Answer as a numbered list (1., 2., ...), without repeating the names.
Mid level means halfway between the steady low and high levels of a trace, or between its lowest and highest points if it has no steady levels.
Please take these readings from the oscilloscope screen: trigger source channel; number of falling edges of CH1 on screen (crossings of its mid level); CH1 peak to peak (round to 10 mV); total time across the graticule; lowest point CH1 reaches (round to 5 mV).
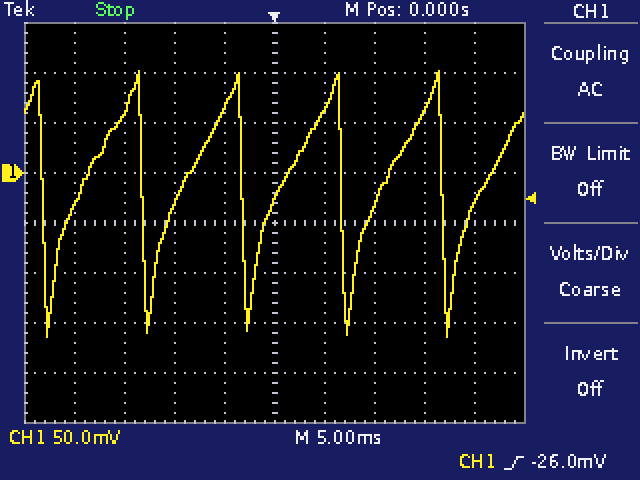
1. CH1
2. 5
3. 270 mV
4. 50 ms
5. -165 mV
